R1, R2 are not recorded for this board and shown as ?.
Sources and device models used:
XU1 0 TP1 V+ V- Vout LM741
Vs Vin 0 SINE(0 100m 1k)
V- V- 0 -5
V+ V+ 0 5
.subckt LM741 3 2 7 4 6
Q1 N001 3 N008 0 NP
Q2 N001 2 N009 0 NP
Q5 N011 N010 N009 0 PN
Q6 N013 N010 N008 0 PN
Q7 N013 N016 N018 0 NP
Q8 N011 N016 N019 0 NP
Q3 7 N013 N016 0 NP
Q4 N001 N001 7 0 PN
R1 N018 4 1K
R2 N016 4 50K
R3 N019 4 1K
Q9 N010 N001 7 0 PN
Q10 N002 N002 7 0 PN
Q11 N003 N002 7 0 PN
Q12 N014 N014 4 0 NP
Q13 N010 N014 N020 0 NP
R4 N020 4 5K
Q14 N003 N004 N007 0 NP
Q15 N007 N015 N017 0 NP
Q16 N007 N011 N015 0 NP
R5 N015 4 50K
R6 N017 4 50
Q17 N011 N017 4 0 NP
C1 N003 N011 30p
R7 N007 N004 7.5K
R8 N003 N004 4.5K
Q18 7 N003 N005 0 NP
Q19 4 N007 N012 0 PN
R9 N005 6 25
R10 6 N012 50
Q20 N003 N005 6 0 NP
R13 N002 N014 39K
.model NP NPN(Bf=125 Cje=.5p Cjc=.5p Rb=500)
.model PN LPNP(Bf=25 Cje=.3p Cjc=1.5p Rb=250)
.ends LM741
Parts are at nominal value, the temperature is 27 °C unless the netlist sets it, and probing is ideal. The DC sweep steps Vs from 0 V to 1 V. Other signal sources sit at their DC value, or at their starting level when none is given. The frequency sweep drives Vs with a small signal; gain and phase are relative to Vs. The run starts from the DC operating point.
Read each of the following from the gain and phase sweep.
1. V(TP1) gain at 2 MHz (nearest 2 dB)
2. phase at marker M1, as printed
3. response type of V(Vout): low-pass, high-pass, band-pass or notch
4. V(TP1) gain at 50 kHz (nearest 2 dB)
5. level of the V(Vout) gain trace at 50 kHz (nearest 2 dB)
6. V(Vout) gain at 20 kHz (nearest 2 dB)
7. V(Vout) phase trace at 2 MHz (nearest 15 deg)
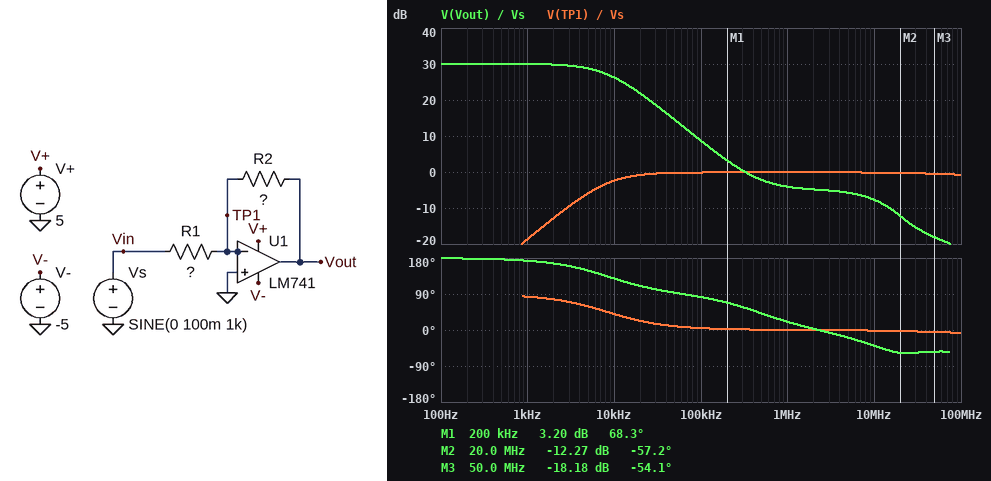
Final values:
0 dB
68.3 deg
low-pass
0 dB
14 dB
22 dB
0 deg
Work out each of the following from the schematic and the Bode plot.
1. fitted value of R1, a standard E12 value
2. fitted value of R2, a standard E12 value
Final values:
470 Ω
15 kΩ
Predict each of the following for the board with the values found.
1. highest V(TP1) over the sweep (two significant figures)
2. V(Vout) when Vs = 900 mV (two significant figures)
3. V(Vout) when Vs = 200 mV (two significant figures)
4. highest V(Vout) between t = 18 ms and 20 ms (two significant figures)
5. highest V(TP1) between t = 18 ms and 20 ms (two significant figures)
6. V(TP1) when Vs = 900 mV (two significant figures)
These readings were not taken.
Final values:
860 mV
-3.5 V
-3.5 V
3.2 V
6.9 mV
770 mV
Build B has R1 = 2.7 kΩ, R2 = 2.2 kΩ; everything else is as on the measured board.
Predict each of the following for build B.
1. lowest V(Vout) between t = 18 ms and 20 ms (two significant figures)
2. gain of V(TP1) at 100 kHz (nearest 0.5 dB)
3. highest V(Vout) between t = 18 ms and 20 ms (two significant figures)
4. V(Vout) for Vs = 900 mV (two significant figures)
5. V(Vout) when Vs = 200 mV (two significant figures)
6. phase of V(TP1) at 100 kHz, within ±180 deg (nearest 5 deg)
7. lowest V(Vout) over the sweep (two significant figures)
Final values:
-81 mV
-2.0 dB
82 mV
-730 mV
-160 mV
30 deg
-810 mV
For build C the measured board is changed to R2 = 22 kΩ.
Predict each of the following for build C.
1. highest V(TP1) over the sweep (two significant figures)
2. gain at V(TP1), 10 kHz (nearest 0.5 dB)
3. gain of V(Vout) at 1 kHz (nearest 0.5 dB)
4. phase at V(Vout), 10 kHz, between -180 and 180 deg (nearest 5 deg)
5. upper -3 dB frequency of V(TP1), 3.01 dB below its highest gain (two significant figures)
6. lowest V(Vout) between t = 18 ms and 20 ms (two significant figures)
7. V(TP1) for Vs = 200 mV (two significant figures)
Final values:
910 mV
-2.0 dB
33.5 dB
125 deg
530 MHz
-3.5 V
120 mV
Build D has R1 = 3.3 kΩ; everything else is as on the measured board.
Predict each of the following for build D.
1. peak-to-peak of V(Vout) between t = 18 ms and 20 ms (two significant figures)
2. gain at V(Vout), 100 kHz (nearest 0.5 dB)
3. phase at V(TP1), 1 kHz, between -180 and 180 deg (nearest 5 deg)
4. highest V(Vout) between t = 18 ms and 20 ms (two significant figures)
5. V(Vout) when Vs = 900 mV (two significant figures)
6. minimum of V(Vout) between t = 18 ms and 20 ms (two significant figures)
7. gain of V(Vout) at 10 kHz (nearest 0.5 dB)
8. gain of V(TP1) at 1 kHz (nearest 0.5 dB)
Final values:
910 mV
6.5 dB
90 deg
460 mV
-3.5 V
-450 mV
13.0 dB
-35.0 dB
